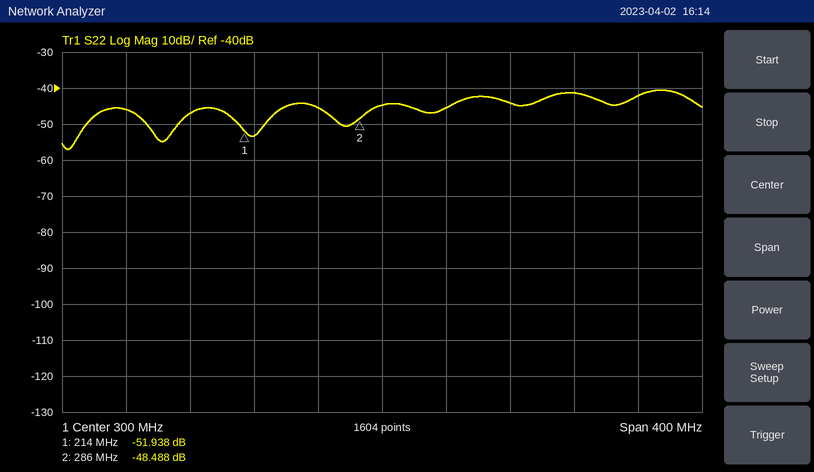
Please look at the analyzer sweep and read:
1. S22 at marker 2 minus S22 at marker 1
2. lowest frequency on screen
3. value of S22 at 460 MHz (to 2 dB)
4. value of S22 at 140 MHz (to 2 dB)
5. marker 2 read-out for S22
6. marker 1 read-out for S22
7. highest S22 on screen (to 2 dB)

3.450 dB
100 MHz
-42 dB
-46 dB
-48.488 dB
-51.938 dB
-40 dB
